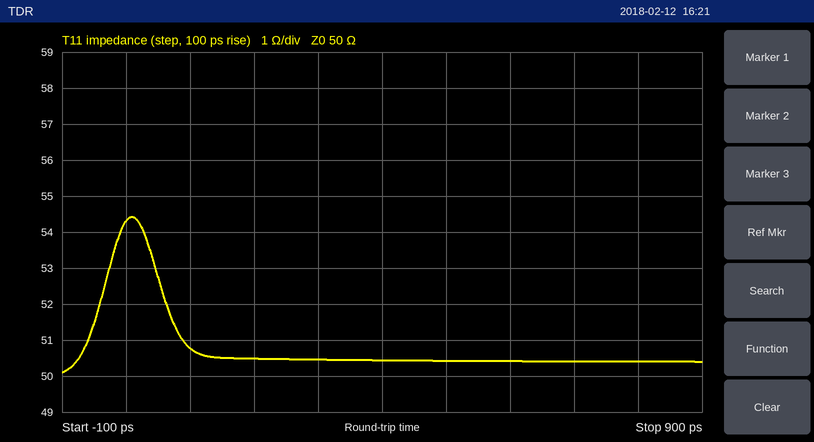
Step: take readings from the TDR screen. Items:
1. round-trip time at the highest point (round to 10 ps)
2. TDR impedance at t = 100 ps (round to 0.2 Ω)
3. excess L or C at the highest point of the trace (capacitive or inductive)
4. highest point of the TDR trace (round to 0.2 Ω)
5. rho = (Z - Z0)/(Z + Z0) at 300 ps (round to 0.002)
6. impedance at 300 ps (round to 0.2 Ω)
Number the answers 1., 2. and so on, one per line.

1. 10 ps
2. 50.8 Ω
3. inductive
4. 54.4 Ω
5. +0.004
6. 50.4 Ω
